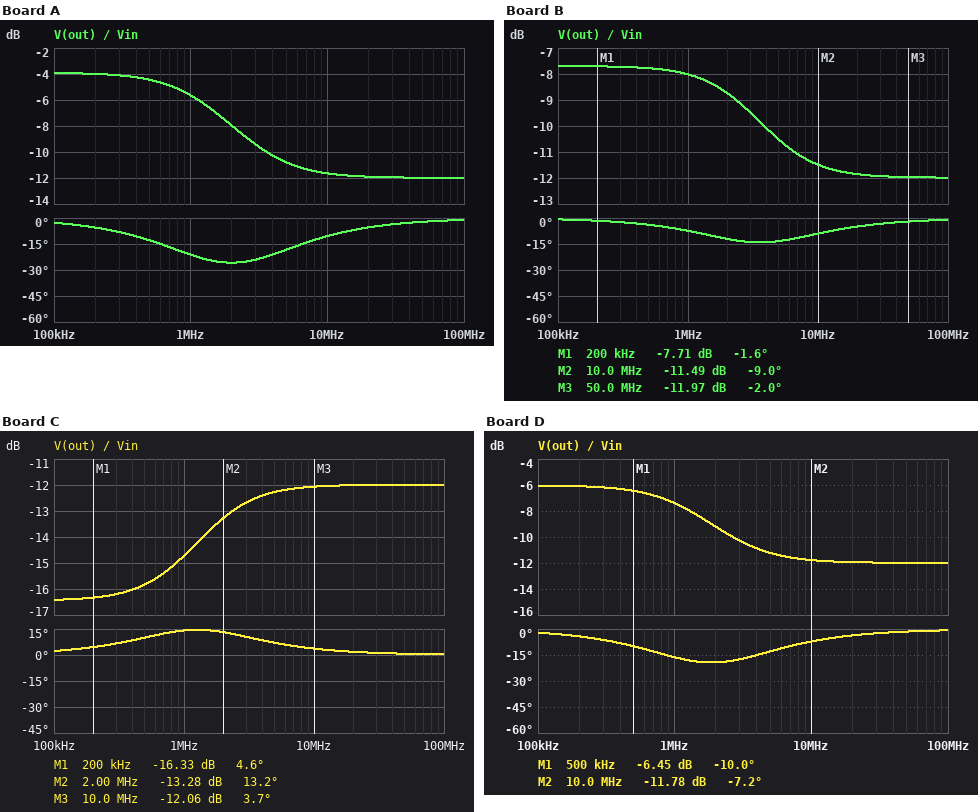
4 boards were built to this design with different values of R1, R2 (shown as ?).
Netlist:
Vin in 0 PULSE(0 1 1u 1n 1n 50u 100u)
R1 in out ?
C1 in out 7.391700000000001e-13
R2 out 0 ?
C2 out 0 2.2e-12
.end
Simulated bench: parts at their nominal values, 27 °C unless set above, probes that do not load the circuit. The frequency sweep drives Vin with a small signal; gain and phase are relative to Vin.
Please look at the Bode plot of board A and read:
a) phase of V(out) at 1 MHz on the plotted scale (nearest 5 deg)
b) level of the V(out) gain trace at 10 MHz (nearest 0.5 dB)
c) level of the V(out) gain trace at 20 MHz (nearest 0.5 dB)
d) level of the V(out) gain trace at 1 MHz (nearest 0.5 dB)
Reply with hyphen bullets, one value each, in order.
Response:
- -20 deg
- -11.5 dB
- -12.0 dB
- -5.5 dB
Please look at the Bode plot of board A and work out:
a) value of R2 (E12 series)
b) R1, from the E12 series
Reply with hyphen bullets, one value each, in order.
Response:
- 120 kΩ
- 68 kΩ
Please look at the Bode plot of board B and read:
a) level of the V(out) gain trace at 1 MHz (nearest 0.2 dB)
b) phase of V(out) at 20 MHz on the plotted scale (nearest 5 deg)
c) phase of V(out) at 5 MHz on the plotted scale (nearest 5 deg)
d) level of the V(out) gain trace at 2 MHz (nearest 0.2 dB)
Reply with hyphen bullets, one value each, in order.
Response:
- -8.0 dB
- -5 deg
- -15 deg
- -8.8 dB
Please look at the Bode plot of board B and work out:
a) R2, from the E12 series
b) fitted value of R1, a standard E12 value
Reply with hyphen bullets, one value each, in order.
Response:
- 33 kΩ
- 47 kΩ
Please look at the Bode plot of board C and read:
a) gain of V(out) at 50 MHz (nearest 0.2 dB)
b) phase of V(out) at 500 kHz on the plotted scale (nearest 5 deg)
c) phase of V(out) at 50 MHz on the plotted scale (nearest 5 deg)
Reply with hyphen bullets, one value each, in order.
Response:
- -12.0 dB
- 10 deg
- 0 deg
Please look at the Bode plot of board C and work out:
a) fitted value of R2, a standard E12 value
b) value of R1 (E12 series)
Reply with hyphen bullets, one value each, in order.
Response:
- 39 kΩ
- 220 kΩ
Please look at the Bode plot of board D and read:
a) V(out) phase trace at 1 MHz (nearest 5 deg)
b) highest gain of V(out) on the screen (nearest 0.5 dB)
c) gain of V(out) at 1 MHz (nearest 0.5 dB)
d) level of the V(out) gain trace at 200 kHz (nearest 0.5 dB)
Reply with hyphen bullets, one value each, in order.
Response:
- -15 deg
- -6.0 dB
- -7.5 dB
- -6.0 dB
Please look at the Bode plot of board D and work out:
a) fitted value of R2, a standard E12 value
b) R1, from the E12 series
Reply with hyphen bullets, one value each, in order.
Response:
- 82 kΩ
- 82 kΩ
